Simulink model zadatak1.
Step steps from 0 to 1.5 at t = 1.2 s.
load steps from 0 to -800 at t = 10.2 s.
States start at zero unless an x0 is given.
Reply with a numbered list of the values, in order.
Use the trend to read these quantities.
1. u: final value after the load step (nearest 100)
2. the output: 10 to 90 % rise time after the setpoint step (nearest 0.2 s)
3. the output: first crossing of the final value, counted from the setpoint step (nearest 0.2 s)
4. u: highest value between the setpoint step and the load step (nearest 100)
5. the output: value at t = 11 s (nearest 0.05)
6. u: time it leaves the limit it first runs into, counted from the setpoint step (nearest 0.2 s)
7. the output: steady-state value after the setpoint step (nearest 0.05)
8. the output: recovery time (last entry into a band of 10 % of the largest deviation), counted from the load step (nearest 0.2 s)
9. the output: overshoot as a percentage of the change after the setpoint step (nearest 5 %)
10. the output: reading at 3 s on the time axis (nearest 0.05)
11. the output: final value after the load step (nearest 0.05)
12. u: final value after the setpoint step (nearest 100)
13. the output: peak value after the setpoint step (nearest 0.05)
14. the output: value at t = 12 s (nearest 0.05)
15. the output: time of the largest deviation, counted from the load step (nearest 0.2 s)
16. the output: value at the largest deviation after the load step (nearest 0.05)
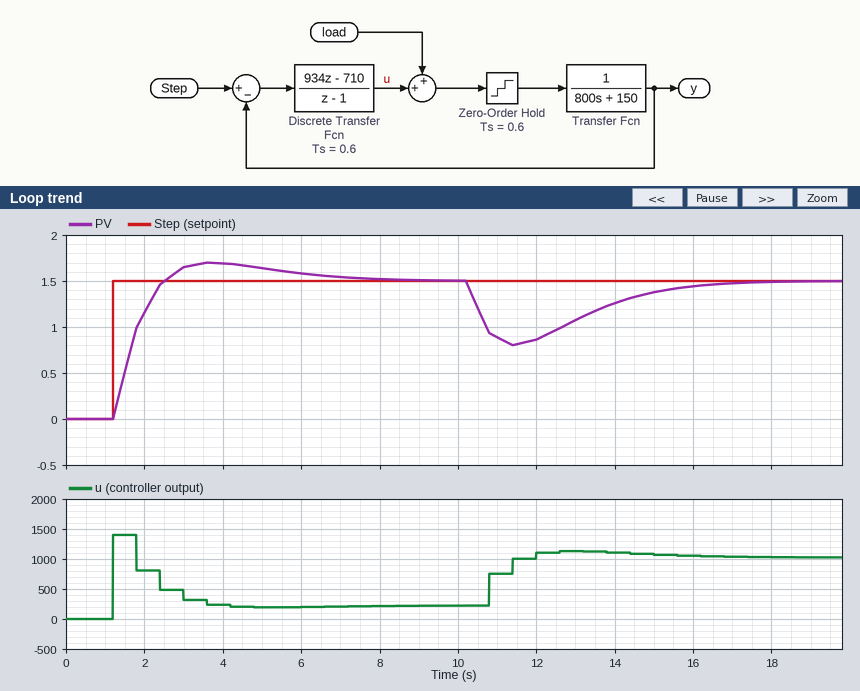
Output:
1. 1000
2. 1.0 s
3. 1.4 s
4. 1400
5. 0.90
6. 0.6 s
7. 1.50
8. 5.6 s
9. 15 %
10. 1.65
11. 1.50
12. 200
13. 1.70
14. 0.85
15. 1.2 s
16. 0.80
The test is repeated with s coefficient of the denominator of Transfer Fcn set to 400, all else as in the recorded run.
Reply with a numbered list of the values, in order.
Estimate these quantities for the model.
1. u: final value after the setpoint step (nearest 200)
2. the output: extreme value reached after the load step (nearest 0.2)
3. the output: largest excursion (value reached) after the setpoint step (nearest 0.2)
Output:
1. 200
2. 0.4
3. 1.8
